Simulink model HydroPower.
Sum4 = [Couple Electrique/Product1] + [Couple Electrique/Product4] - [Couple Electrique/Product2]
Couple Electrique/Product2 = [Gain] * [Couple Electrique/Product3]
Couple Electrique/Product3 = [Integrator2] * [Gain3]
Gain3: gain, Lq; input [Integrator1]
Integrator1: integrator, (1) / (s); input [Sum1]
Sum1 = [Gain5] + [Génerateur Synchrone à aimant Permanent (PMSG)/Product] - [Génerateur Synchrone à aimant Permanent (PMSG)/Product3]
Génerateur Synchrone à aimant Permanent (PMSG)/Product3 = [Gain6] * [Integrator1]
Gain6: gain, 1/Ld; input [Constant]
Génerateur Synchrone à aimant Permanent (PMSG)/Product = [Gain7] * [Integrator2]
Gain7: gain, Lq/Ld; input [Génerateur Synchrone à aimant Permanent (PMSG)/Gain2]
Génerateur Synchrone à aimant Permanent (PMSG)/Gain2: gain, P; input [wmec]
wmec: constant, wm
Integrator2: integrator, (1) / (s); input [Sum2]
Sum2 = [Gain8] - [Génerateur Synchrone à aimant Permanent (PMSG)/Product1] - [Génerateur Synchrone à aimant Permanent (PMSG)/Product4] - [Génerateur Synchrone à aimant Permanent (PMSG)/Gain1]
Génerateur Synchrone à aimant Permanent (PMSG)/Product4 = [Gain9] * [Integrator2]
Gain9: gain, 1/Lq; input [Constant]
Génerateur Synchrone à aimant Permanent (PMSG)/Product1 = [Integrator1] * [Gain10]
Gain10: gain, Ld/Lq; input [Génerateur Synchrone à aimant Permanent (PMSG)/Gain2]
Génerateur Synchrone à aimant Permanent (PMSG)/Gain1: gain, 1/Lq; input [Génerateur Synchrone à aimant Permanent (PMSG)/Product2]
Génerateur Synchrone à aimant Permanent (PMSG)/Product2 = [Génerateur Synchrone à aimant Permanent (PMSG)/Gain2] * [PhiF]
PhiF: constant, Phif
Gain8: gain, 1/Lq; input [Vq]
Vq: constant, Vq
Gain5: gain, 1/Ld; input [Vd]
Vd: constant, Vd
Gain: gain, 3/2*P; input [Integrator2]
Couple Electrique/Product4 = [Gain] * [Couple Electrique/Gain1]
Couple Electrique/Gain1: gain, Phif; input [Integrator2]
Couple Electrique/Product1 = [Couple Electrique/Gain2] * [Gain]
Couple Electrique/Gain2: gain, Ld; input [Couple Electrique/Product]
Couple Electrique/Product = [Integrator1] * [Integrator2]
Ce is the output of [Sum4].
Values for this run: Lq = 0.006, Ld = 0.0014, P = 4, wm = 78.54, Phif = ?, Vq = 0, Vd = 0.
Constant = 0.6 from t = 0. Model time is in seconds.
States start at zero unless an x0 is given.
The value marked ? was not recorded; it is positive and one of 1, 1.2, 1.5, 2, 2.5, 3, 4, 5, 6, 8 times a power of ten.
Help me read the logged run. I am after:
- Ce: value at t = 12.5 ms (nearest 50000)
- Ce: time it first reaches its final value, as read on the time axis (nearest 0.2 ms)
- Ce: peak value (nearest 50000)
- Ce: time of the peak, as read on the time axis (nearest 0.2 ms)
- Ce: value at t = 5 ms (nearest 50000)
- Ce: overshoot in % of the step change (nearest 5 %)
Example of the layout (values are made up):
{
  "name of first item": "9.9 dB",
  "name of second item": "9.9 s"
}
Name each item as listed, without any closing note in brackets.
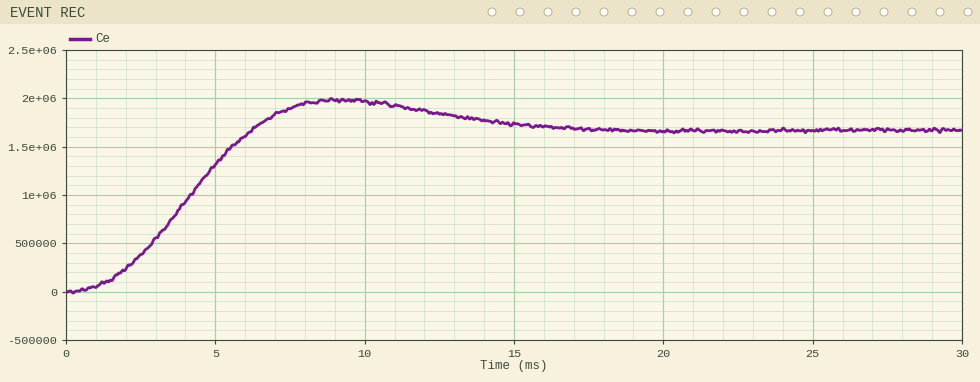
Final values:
{
  "Ce: value at t = 12.5 ms": "1850000",
  "Ce: time it first reaches its final value, as read on the time axis": "6.2 ms",
  "Ce: peak value": "2000000",
  "Ce: time of the peak, as read on the time axis": "9.2 ms",
  "Ce: value at t = 5 ms": "1300000",
  "Ce: overshoot in % of the step change": "20 %"
}
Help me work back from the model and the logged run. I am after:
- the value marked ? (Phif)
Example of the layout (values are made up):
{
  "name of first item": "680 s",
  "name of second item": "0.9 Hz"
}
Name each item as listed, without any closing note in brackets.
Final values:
{
  "the value marked ?": "1.5"
}
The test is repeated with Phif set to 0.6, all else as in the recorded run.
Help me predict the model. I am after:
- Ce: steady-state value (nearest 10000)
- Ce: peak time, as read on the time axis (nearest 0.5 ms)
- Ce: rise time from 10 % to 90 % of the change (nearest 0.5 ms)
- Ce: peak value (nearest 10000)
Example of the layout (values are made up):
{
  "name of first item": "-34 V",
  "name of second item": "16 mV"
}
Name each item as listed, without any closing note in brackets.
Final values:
{
  "Ce: steady-state value": "110000",
  "Ce: peak time, as read on the time axis": "9.0 ms",
  "Ce: rise time from 10 % to 90 % of the change": "4.0 ms",
  "Ce: peak value": "130000"
}
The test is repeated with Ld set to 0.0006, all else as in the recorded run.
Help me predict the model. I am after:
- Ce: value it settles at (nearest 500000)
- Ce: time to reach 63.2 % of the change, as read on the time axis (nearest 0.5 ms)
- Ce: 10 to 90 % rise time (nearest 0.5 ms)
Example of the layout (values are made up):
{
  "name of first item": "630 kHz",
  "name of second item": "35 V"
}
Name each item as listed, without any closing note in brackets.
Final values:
{
  "Ce: value it settles at": "7500000",
  "Ce: time to reach 63.2 % of the change, as read on the time axis": "9.0 ms",
  "Ce: 10 to 90 % rise time": "12.0 ms"
}
